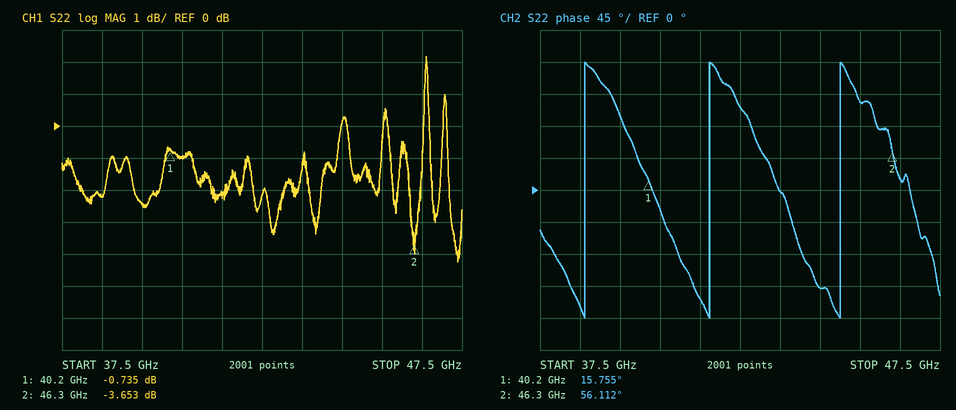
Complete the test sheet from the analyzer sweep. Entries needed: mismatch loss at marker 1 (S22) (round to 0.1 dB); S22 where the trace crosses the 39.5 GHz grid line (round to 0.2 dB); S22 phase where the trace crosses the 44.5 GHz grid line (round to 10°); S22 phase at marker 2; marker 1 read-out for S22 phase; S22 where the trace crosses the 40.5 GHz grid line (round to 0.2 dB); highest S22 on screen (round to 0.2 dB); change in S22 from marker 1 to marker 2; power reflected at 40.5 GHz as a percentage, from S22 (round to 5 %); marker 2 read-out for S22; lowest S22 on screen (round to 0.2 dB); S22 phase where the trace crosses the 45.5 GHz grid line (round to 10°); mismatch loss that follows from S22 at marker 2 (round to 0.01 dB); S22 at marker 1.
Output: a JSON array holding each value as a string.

["8.1 dB", "-2.4 dB", "-140°", "56.112°", "15.755°", "-1.0 dB", "2.2 dB", "-2.918 dB", "80 %", "-3.653 dB", "-4.2 dB", "120°", "2.45 dB", "-0.735 dB"]
